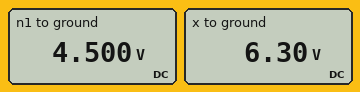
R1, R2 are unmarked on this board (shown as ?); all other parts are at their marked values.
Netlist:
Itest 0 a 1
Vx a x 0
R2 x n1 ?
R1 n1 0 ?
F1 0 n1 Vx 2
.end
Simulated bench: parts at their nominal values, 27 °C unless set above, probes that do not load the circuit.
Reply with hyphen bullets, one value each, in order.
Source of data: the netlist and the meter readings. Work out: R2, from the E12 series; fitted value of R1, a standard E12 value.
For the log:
- 1.8 Ω
- 1.5 Ω
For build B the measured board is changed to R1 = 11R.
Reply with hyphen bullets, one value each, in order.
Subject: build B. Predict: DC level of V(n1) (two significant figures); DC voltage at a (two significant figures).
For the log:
- 33 V
- 35 V
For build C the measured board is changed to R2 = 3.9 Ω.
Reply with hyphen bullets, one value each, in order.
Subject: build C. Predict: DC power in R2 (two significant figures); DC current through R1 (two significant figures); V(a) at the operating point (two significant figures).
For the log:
- 3.9 W
- 3.0 A
- 8.4 V
